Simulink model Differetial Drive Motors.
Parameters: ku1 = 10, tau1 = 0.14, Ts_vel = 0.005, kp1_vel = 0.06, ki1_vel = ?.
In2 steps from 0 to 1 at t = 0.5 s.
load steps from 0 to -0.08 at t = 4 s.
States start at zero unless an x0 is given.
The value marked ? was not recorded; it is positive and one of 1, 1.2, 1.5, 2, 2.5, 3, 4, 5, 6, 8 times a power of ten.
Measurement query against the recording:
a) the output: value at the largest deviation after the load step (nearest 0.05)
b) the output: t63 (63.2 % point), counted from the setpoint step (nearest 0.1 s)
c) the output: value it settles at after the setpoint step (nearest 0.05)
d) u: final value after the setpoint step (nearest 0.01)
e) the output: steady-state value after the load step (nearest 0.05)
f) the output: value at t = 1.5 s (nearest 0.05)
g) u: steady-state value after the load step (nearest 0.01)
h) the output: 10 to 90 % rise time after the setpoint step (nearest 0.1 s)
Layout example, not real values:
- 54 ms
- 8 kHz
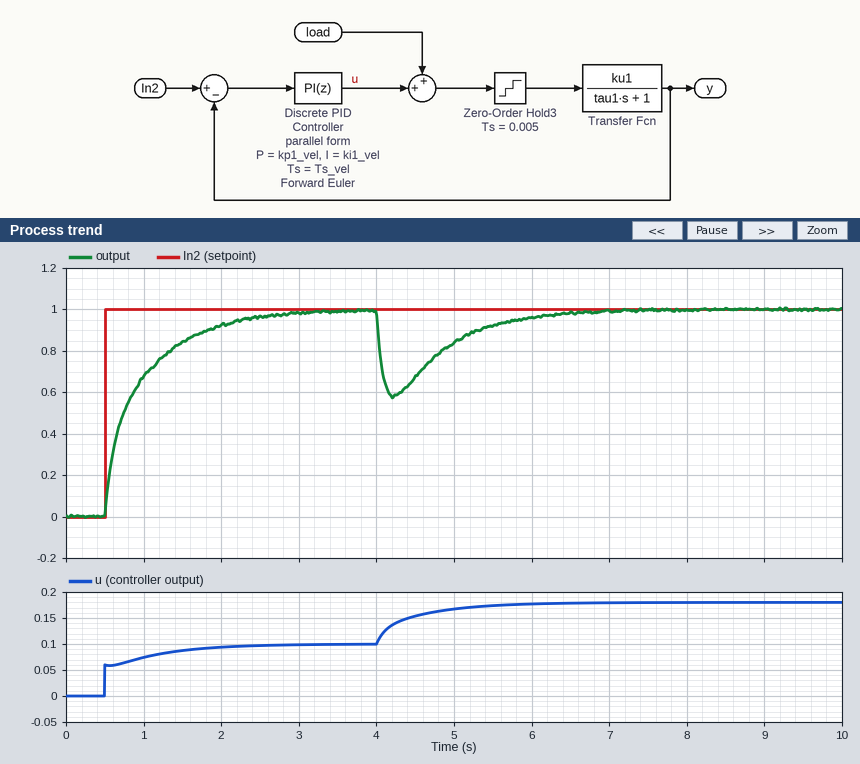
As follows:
- 0.60
- 0.4 s
- 1.00
- 0.10
- 1.00
- 0.85
- 0.18
- 1.3 s
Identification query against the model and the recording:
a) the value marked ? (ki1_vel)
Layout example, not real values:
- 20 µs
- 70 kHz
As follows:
- 0.2
